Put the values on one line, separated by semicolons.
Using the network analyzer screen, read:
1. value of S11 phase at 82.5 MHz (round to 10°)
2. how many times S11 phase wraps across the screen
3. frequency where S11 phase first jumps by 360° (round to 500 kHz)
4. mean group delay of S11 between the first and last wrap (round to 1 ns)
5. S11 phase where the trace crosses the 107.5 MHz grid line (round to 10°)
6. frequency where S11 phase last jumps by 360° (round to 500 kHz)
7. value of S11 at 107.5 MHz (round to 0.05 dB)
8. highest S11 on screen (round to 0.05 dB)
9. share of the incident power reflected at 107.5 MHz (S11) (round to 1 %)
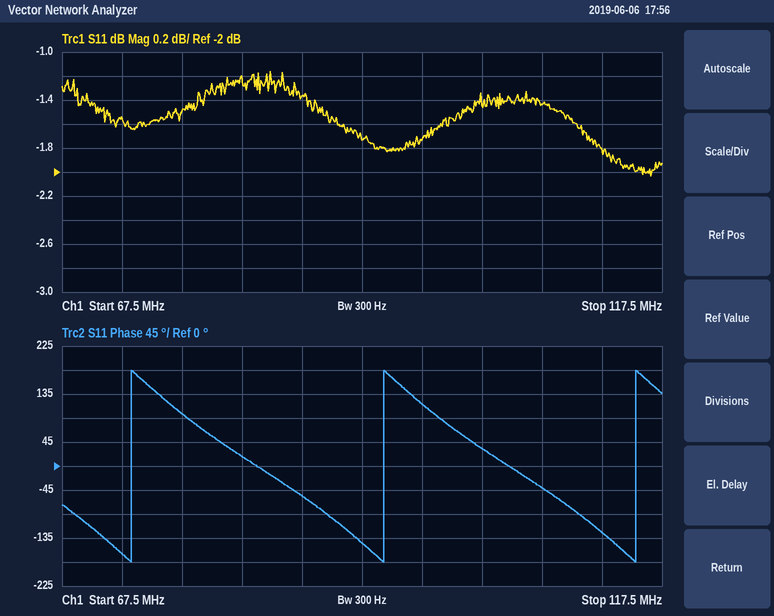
20°; 3; 73.5 MHz; 48 ns; -40°; 115.5 MHz; -1.45 dB; -1.15 dB; 72 %
